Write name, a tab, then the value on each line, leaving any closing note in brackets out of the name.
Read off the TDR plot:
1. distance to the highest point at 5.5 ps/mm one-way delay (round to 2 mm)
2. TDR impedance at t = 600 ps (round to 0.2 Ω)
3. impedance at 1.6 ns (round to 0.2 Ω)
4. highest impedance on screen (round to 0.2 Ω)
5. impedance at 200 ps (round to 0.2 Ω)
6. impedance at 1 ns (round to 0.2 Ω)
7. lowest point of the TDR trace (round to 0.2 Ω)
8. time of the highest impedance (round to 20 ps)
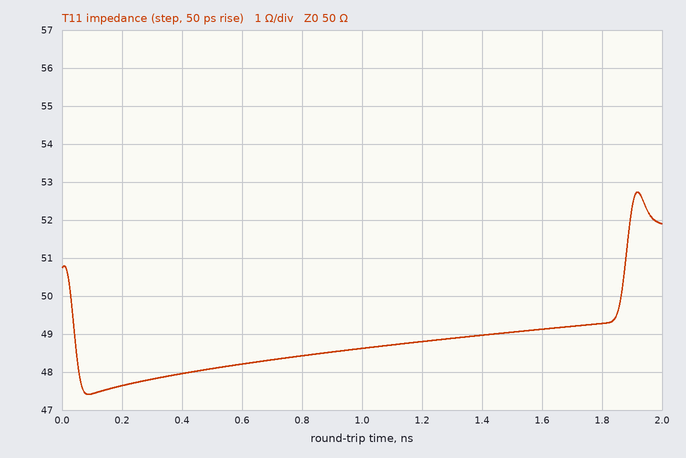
distance to the highest point at 5.5 ps/mm one-way delay	174 mm
TDR impedance at t = 600 ps	48.2 Ω
impedance at 1.6 ns	49.2 Ω
highest impedance on screen	52.8 Ω
impedance at 200 ps	47.6 Ω
impedance at 1 ns	48.6 Ω
lowest point of the TDR trace	47.4 Ω
time of the highest impedance	1.92 ns
